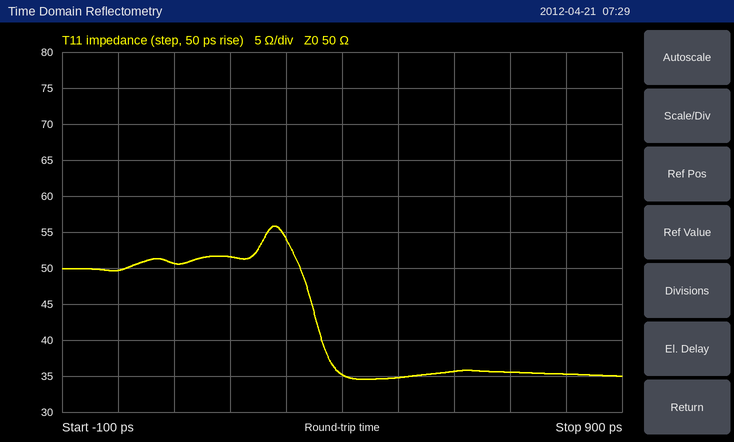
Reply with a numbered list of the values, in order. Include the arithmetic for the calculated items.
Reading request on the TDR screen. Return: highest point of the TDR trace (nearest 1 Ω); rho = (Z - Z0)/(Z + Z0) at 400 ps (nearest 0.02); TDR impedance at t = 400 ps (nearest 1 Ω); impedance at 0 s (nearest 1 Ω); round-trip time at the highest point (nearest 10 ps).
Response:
1. 56 Ω
2. (35 − 50)/(35 + 50) ≈ -0.18
3. 35 Ω
4. 50 Ω
5. 280 ps
